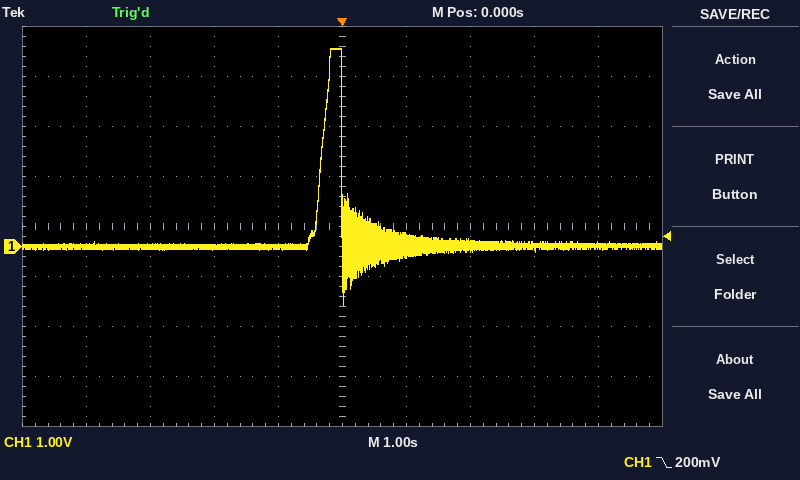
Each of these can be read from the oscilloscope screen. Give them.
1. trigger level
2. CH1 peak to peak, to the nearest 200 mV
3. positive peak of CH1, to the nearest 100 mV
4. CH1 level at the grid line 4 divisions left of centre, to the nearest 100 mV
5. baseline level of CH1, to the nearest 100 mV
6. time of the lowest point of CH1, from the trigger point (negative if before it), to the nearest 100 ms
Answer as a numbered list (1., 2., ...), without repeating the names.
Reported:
1. 200 mV
2. 5.2 V
3. 4.0 V
4. 0.0 V
5. 0.0 V
6. 0.0 s
